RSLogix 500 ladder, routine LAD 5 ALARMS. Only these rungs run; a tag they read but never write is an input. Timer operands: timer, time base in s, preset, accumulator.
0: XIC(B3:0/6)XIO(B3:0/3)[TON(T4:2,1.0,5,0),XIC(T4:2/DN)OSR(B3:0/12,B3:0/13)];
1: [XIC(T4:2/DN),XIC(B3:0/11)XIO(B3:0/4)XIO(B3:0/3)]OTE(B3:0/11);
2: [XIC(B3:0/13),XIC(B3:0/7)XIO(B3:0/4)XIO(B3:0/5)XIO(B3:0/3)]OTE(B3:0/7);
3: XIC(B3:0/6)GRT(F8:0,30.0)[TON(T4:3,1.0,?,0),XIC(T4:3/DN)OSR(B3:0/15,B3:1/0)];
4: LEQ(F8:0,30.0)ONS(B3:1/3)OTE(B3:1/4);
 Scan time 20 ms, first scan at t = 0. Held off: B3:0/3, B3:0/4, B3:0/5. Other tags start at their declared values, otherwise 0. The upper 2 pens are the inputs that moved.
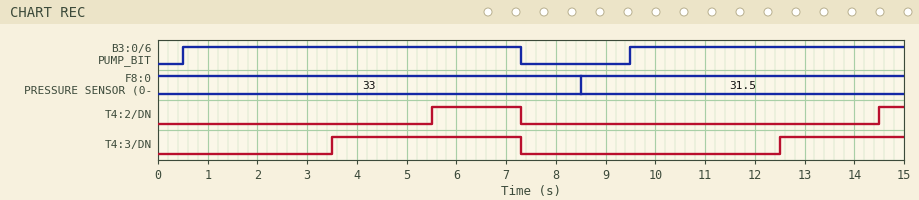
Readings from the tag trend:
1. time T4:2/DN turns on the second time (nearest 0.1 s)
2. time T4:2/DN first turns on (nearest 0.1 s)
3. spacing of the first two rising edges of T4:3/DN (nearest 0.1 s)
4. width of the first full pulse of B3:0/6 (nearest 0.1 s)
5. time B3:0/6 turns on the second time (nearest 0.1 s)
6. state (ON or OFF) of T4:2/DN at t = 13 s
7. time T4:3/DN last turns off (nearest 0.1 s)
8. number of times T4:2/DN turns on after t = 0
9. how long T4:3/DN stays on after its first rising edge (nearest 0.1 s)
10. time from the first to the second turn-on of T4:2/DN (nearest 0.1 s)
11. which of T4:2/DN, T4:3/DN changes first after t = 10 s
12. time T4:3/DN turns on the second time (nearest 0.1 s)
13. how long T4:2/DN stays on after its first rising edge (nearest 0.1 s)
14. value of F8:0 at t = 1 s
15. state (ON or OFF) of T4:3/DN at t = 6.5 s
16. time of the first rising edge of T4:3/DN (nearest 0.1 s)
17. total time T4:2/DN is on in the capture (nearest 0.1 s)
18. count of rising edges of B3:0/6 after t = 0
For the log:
14.5 s
5.5 s
9.0 s
6.8 s
9.5 s
OFF
7.3 s
2
3.8 s
9.0 s
T4:3/DN
12.5 s
1.8 s
33
ON
3.5 s
2.3 s
2
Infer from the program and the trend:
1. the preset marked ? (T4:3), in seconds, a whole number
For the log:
3 s
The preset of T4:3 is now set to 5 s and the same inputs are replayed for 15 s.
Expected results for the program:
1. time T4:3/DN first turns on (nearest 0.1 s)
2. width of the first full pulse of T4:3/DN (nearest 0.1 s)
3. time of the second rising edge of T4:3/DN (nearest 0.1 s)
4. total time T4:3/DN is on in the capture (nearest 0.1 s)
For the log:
5.5 s
1.8 s
14.5 s
2.3 s
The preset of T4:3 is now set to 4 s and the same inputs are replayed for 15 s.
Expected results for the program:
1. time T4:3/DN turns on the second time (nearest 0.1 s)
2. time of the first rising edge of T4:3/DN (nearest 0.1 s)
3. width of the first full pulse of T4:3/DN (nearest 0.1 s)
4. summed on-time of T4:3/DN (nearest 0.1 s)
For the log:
13.5 s
4.5 s
2.8 s
4.3 s
